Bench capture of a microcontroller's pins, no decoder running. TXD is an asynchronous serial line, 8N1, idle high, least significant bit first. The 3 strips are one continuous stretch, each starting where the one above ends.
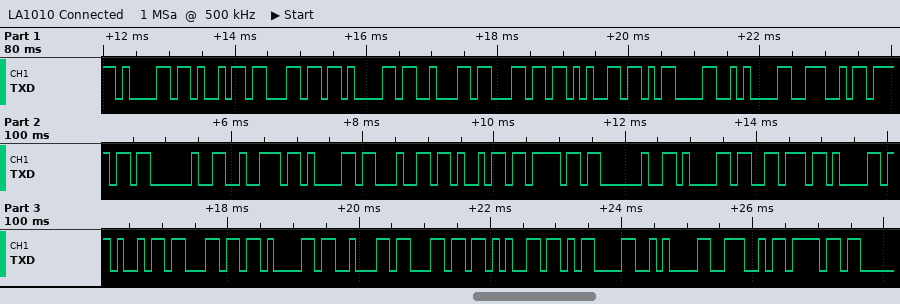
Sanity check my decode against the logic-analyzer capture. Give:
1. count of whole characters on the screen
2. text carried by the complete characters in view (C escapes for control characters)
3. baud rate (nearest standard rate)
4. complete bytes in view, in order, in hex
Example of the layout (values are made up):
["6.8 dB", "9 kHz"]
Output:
["31", "\"ailable\\r\\nNo radio available\\r\\nNo\"", "9600 baud", "61 69 6C 61 62 6C 65 0D 0A 4E 6F 20 72 61 64 69 6F 20 61 76 61 69 6C 61 62 6C 65 0D 0A 4E 6F"]
